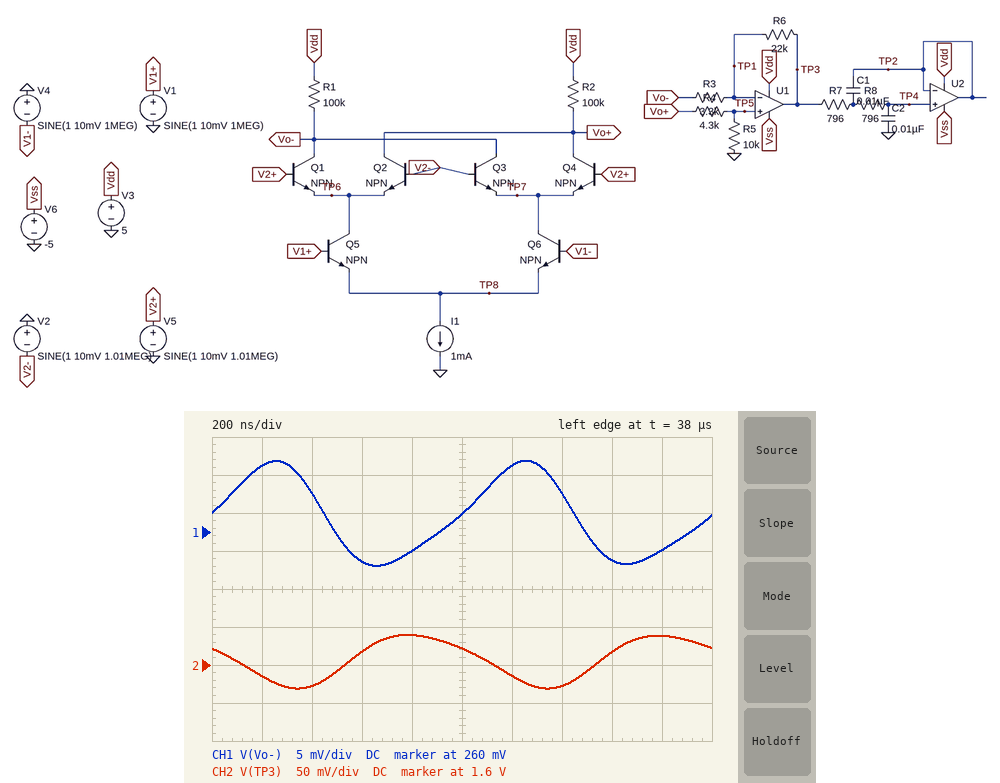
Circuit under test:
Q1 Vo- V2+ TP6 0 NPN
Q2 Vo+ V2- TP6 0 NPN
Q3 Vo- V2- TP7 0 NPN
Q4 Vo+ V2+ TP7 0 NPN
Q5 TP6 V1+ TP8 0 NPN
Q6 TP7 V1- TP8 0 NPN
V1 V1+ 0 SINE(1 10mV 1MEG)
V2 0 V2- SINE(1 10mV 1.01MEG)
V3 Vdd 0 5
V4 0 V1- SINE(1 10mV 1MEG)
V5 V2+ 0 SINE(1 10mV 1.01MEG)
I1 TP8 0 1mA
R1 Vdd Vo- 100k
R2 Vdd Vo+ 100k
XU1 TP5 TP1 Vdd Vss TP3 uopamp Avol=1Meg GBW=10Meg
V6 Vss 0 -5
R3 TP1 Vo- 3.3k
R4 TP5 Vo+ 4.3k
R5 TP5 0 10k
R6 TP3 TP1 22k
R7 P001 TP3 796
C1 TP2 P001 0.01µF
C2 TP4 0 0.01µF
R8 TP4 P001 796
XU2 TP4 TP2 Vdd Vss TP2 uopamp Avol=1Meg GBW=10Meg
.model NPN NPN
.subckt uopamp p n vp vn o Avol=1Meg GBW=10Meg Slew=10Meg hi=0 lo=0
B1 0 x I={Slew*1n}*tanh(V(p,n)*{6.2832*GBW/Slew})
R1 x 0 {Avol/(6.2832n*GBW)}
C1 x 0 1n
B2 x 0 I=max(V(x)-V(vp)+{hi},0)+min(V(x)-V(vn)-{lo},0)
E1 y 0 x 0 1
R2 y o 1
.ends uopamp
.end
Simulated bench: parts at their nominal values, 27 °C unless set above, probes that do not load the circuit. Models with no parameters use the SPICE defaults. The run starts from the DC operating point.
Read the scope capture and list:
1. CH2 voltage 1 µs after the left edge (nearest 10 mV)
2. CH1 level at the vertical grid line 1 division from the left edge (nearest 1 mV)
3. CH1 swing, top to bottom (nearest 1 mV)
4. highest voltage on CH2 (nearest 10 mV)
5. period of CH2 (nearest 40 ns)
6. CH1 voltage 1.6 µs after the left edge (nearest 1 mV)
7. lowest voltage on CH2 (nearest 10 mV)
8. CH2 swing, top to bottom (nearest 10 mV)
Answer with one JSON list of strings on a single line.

["1.62 V", "269 mV", "14 mV", "1.64 V", "1.00 µs", "256 mV", "1.57 V", "70 mV"]
